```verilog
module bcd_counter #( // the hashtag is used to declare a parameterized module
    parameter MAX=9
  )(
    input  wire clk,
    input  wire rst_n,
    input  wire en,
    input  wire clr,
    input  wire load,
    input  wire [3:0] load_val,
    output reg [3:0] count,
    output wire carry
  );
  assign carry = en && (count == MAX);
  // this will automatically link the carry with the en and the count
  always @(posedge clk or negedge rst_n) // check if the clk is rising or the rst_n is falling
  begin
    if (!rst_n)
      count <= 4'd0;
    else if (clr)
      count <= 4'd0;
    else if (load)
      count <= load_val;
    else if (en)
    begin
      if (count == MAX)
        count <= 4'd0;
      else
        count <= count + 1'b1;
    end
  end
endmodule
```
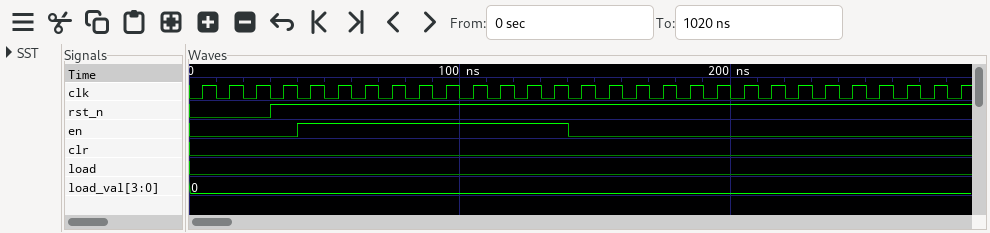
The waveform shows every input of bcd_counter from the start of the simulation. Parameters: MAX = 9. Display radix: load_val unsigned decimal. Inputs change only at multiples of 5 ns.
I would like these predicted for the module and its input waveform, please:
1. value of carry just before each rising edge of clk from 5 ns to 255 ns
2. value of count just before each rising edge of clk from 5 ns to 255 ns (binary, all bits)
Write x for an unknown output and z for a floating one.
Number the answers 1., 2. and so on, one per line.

1. 0 0 0 0 0 0 0 0 0 0 0 0 0 1 0 0 0 0 0 0 0 0 0 0 0 0
2. 0000, 0000, 0000, 0000, 0000, 0001, 0010, 0011, 0100, 0101, 0110, 0111, 1000, 1001, 0000, 0000, 0000, 0000, 0000, 0000, 0000, 0000, 0000, 0000, 0000, 0000
